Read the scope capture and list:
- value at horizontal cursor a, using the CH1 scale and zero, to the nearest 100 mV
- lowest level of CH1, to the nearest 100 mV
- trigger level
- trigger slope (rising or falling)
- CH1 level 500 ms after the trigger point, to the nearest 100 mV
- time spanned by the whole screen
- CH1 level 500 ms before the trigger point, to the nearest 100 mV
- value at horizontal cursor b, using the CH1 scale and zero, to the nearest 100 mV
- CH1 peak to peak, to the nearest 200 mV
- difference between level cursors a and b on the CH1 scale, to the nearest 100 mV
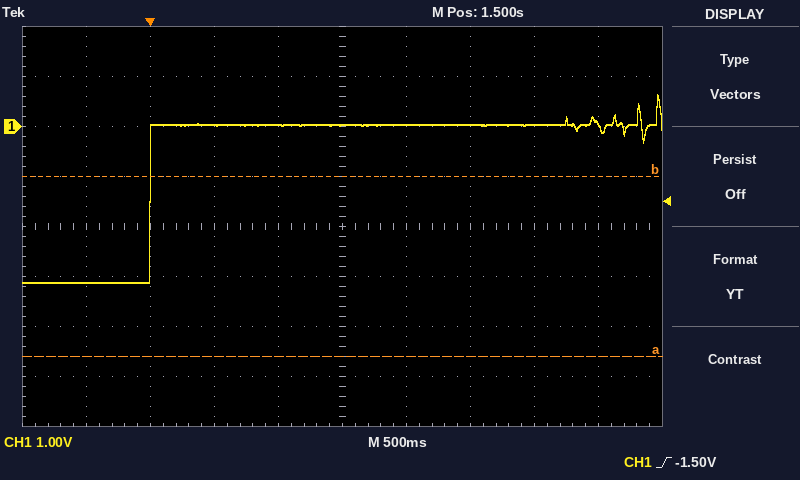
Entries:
-4.6 V
-3.1 V
-1.50 V
rising
0.0 V
5 s
-3.1 V
-1.0 V
3.8 V
3.6 V
